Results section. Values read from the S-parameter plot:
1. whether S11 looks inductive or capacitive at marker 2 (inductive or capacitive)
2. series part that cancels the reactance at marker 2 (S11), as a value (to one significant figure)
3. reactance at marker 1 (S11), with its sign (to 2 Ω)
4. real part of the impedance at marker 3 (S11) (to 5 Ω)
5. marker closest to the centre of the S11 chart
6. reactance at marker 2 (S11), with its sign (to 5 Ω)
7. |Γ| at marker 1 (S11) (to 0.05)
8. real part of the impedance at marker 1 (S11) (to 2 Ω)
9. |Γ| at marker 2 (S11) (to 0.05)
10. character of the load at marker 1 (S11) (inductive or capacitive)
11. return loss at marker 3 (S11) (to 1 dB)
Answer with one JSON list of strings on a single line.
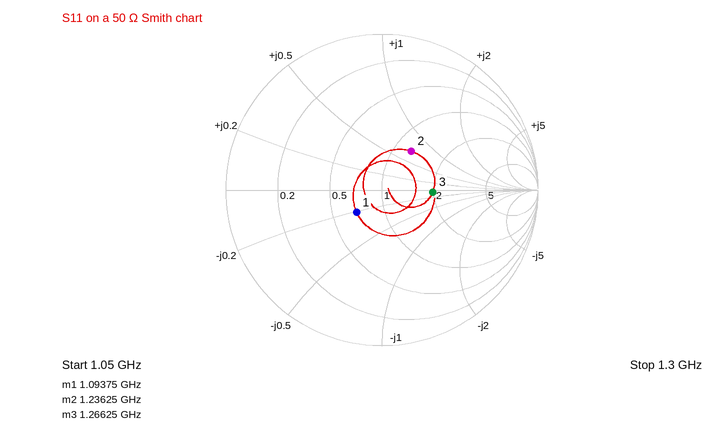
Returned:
["inductive", "4 pF", "-10 Ω", "100 Ω", "marker 1", "+35 Ω", "0.20", "34 Ω", "0.30", "capacitive", "10 dB"]
